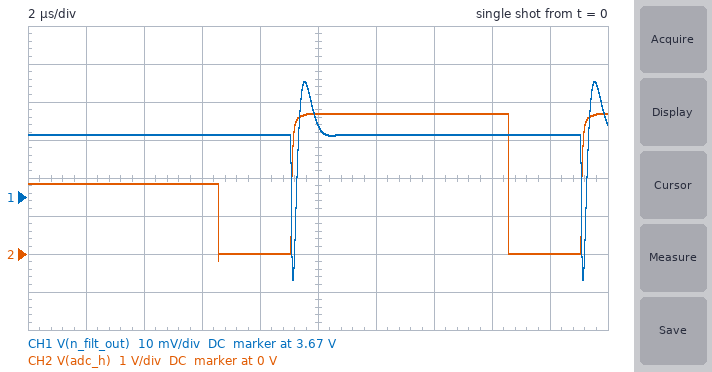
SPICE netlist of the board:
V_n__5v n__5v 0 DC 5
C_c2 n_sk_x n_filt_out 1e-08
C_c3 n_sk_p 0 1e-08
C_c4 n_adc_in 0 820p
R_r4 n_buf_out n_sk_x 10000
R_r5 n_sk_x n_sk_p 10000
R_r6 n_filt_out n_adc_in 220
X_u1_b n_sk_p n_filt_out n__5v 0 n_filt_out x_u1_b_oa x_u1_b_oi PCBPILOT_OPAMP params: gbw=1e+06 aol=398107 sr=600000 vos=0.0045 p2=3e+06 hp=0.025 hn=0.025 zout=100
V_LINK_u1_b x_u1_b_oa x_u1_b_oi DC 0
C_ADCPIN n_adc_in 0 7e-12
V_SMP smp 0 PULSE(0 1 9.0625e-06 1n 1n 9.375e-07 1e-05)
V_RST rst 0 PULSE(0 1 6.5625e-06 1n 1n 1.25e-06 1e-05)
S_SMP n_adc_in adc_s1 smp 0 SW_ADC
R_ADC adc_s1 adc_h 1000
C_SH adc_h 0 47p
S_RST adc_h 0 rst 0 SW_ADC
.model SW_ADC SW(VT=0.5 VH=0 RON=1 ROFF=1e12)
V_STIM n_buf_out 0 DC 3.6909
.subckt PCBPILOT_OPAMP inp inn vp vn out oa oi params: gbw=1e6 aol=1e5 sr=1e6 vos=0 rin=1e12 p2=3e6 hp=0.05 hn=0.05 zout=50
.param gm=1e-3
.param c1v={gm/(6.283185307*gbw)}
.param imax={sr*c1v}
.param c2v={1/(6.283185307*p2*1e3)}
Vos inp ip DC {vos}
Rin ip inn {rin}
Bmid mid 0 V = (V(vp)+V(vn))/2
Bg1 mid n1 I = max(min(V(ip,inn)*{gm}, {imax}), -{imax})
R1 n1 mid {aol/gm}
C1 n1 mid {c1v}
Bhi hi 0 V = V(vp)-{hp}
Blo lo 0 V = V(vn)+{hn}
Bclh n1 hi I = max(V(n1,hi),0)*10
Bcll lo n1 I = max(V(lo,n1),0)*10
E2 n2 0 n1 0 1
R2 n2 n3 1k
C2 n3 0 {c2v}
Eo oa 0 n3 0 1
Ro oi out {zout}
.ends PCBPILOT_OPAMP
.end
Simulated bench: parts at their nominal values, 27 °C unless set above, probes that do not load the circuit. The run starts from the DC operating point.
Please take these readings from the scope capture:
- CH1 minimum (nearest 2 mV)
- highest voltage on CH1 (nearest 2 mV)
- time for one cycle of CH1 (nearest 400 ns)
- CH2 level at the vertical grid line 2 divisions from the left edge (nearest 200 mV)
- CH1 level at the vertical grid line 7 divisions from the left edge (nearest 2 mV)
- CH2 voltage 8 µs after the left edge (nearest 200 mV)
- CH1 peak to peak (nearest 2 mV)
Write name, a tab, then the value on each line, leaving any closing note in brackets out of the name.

CH1 minimum	3.648 V
highest voltage on CH1	3.700 V
time for one cycle of CH1	10.0 µs
CH2 level at the vertical grid line 2 divisions from the left edge	1.8 V
CH1 level at the vertical grid line 7 divisions from the left edge	3.686 V
CH2 voltage 8 µs after the left edge	0 V
CH1 peak to peak	52 mV
